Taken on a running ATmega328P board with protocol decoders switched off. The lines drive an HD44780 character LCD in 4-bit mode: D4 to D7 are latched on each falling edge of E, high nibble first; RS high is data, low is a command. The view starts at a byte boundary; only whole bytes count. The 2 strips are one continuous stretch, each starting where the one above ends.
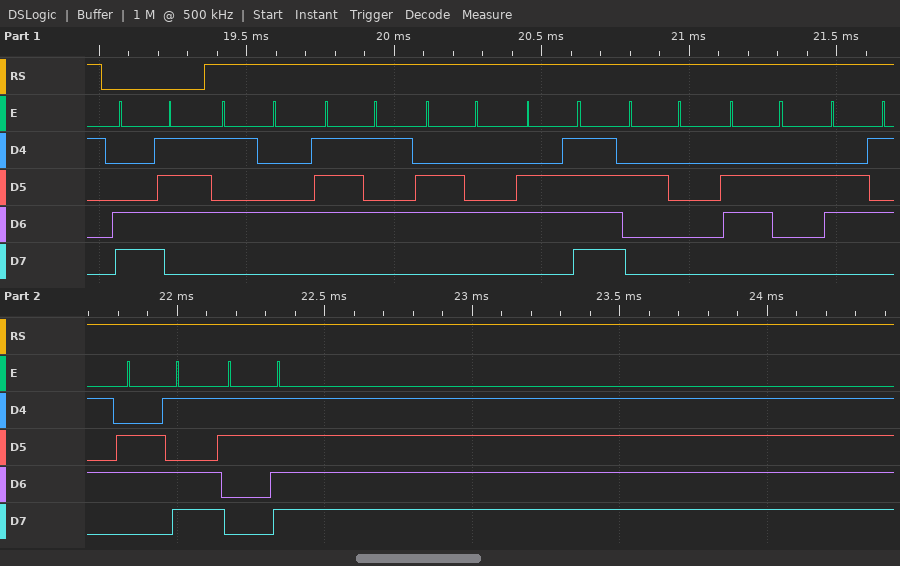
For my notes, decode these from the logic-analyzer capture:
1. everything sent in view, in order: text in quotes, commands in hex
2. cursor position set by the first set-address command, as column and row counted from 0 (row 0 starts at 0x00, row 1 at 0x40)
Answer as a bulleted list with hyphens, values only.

- 0xC7 "Tudo bem?"
- column 7, row 1
